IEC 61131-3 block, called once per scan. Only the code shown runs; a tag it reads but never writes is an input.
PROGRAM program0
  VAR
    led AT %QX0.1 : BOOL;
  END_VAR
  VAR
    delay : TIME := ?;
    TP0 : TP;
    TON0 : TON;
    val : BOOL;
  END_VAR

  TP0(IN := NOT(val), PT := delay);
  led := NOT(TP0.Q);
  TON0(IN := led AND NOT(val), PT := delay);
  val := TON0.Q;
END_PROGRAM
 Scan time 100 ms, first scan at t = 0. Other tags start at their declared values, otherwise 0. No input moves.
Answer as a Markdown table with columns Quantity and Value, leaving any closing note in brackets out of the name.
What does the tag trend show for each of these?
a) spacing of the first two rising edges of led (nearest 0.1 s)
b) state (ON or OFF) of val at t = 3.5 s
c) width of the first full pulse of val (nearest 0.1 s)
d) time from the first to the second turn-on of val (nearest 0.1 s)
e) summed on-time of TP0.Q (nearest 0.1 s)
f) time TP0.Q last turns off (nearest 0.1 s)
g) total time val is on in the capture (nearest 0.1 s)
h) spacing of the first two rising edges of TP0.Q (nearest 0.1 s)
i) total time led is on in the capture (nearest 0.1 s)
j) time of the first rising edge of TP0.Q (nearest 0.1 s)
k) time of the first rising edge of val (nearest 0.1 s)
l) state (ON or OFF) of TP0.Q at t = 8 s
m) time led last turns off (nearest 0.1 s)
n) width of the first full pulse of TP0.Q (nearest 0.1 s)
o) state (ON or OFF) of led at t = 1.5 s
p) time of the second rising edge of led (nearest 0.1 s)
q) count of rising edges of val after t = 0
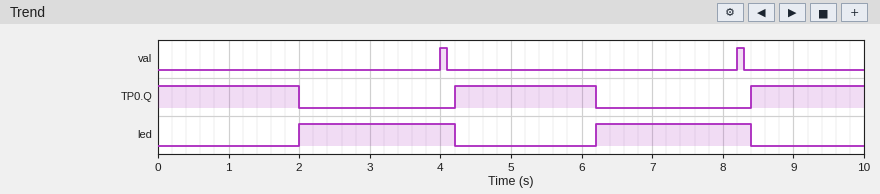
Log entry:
| Quantity | Value |
|---|---|
| spacing of the first two rising edges of led | 4.2 s |
| state (ON or OFF) of val at t = 3.5 s | OFF |
| width of the first full pulse of val | 0.1 s |
| time from the first to the second turn-on of val | 4.2 s |
| summed on-time of TP0.Q | 5.6 s |
| time TP0.Q last turns off | 6.2 s |
| total time val is on in the capture | 0.2 s |
| spacing of the first two rising edges of TP0.Q | 4.2 s |
| total time led is on in the capture | 4.4 s |
| time of the first rising edge of TP0.Q | 4.2 s |
| time of the first rising edge of val | 4.0 s |
| state (ON or OFF) of TP0.Q at t = 8 s | OFF |
| time led last turns off | 8.4 s |
| width of the first full pulse of TP0.Q | 2.0 s |
| state (ON or OFF) of led at t = 1.5 s | OFF |
| time of the second rising edge of led | 6.2 s |
| count of rising edges of val after t = 0 | 2 |
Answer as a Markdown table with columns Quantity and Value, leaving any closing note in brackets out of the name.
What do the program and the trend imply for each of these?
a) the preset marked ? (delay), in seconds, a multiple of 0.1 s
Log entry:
| Quantity | Value |
|---|---|
| the preset marked ? (delay), in seconds, a multiple of 0.1 s | 2.0 s |
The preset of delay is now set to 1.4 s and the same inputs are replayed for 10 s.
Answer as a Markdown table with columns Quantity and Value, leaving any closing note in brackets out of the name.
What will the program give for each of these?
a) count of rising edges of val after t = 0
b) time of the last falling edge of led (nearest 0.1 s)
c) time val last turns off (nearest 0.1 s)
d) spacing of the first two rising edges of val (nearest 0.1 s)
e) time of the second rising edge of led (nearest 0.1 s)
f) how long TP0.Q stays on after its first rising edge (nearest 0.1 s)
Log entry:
| Quantity | Value |
|---|---|
| count of rising edges of val after t = 0 | 3 |
| time of the last falling edge of led | 9.0 s |
| time val last turns off | 8.9 s |
| spacing of the first two rising edges of val | 3.0 s |
| time of the second rising edge of led | 4.4 s |
| how long TP0.Q stays on after its first rising edge | 1.4 s |
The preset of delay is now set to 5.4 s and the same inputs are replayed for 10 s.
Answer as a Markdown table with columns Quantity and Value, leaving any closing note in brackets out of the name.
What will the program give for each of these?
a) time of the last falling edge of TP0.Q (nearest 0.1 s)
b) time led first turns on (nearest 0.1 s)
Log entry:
| Quantity | Value |
|---|---|
| time of the last falling edge of TP0.Q | 5.4 s |
| time led first turns on | 5.4 s |
